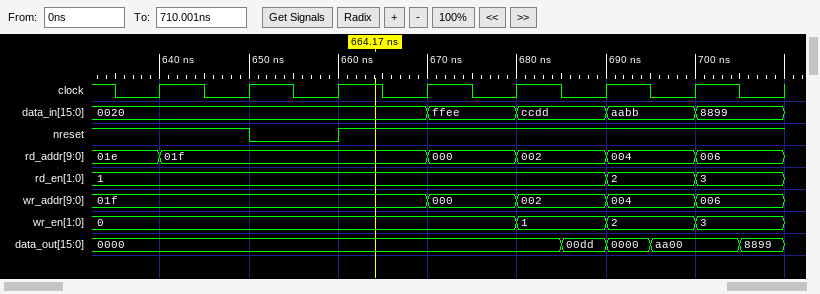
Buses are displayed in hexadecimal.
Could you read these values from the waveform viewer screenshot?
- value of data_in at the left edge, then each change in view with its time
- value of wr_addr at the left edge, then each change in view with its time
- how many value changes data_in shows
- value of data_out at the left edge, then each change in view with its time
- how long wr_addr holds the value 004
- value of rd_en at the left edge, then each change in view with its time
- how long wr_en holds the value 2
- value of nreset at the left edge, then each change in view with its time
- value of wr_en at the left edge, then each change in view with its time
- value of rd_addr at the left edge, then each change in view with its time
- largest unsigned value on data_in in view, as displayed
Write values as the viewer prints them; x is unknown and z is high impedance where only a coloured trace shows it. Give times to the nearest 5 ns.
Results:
0020, ffee at 670 ns, ccdd at 680 ns, aabb at 690 ns, 8899 at 700 ns
01f, 000 at 670 ns, 002 at 680 ns, 004 at 690 ns, 006 at 700 ns
4
0000, 00dd at 685 ns, 0000 at 690 ns, aa00 at 695 ns, 8899 at 705 ns
10 ns
1, 2 at 690 ns, 3 at 700 ns
10 ns
1, 0 at 650 ns, 1 at 660 ns
0, 1 at 680 ns, 2 at 690 ns, 3 at 700 ns
01e, 01f at 640 ns, 000 at 670 ns, 002 at 680 ns, 004 at 690 ns, 006 at 700 ns
ffee
